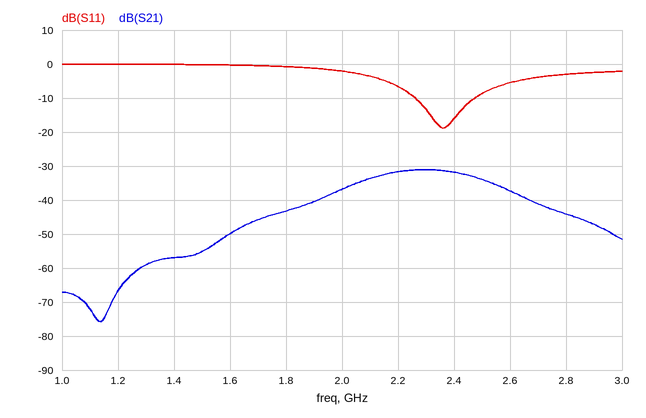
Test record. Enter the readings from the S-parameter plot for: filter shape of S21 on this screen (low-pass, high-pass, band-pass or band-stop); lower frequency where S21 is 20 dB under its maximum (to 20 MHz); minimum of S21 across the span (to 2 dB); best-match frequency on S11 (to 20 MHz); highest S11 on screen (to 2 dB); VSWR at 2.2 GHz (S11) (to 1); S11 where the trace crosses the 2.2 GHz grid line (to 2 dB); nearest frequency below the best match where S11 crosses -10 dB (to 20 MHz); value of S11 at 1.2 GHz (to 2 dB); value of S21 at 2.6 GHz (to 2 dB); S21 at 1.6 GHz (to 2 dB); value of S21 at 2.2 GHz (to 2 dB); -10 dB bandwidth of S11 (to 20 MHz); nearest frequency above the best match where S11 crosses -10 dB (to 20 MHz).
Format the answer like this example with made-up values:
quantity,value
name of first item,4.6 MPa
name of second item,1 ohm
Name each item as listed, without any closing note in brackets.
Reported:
quantity,value
filter shape of S21 on this screen,band-pass
lower frequency where S21 is 20 dB under its maximum,1.58 GHz
minimum of S21 across the span,-76 dB
best-match frequency on S11,2.36 GHz
highest S11 on screen,0 dB
VSWR at 2.2 GHz (S11),3
S11 where the trace crosses the 2.2 GHz grid line,-6 dB
nearest frequency below the best match where S11 crosses -10 dB,2.26 GHz
value of S11 at 1.2 GHz,0 dB
value of S21 at 2.6 GHz,-38 dB
S21 at 1.6 GHz,-50 dB
value of S21 at 2.2 GHz,-32 dB
-10 dB bandwidth of S11,220 MHz
nearest frequency above the best match where S11 crosses -10 dB,2.48 GHz
